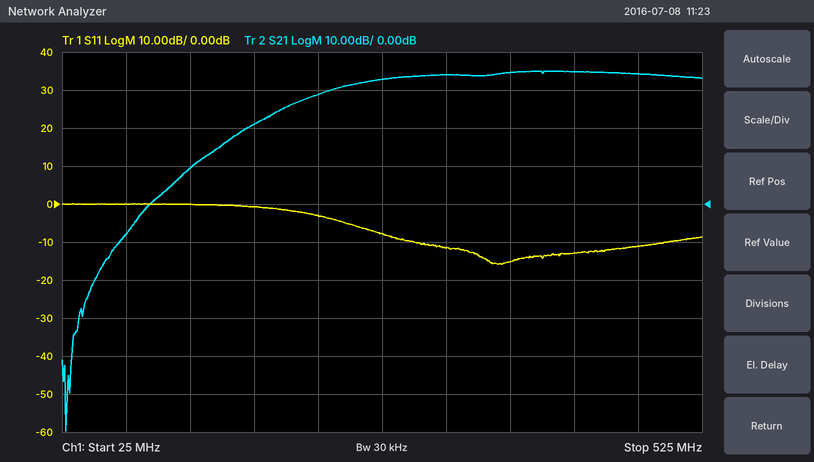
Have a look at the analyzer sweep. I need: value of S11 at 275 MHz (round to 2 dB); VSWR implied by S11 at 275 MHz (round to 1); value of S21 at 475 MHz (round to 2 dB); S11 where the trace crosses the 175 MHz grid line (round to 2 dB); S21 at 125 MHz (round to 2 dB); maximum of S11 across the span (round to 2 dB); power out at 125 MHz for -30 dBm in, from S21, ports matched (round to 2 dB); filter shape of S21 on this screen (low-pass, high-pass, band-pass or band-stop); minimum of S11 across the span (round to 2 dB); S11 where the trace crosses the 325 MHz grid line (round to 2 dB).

-8 dB
2
34 dB
0 dB
10 dB
0 dB
-20 dBm
high-pass
-16 dB
-12 dB
